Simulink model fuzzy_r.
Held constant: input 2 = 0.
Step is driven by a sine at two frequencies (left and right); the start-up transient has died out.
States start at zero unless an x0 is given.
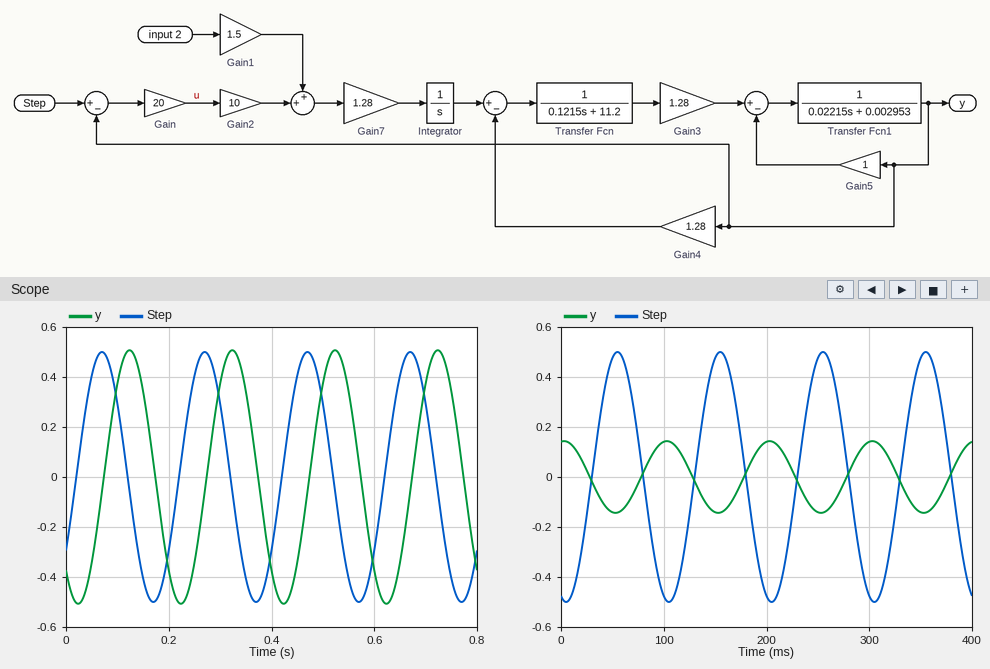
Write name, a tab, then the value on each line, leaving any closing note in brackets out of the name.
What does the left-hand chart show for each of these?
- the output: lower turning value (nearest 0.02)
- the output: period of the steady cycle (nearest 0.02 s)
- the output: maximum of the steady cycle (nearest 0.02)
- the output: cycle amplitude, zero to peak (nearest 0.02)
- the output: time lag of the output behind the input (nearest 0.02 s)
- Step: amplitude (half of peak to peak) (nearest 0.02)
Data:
the output: lower turning value	-0.50
the output: period of the steady cycle	0.20 s
the output: maximum of the steady cycle	0.50
the output: cycle amplitude, zero to peak	0.50
the output: time lag of the output behind the input	0.06 s
Step: amplitude (half of peak to peak)	0.50
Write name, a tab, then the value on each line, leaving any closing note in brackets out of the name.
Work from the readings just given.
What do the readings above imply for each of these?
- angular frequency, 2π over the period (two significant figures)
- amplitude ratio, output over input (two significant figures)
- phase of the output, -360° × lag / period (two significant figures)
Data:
angular frequency, 2π over the period	31 rad/s
amplitude ratio, output over input	1.0
phase of the output, -360° × lag / period	-110°
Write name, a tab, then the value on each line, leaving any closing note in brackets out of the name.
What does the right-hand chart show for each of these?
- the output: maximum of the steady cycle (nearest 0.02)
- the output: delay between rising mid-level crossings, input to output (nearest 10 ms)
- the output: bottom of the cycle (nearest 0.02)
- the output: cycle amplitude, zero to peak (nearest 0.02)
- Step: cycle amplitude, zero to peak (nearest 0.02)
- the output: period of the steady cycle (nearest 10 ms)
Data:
the output: maximum of the steady cycle	0.14
the output: delay between rising mid-level crossings, input to output	50 ms
the output: bottom of the cycle	-0.14
the output: cycle amplitude, zero to peak	0.14
Step: cycle amplitude, zero to peak	0.50
the output: period of the steady cycle	100 ms
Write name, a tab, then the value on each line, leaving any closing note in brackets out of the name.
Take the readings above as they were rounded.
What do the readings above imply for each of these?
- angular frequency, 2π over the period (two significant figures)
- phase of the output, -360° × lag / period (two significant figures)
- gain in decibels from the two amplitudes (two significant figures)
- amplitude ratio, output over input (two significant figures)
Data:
angular frequency, 2π over the period	0.063 rad/ms
phase of the output, -360° × lag / period	-180°
gain in decibels from the two amplitudes	-11 dB
amplitude ratio, output over input	0.28
